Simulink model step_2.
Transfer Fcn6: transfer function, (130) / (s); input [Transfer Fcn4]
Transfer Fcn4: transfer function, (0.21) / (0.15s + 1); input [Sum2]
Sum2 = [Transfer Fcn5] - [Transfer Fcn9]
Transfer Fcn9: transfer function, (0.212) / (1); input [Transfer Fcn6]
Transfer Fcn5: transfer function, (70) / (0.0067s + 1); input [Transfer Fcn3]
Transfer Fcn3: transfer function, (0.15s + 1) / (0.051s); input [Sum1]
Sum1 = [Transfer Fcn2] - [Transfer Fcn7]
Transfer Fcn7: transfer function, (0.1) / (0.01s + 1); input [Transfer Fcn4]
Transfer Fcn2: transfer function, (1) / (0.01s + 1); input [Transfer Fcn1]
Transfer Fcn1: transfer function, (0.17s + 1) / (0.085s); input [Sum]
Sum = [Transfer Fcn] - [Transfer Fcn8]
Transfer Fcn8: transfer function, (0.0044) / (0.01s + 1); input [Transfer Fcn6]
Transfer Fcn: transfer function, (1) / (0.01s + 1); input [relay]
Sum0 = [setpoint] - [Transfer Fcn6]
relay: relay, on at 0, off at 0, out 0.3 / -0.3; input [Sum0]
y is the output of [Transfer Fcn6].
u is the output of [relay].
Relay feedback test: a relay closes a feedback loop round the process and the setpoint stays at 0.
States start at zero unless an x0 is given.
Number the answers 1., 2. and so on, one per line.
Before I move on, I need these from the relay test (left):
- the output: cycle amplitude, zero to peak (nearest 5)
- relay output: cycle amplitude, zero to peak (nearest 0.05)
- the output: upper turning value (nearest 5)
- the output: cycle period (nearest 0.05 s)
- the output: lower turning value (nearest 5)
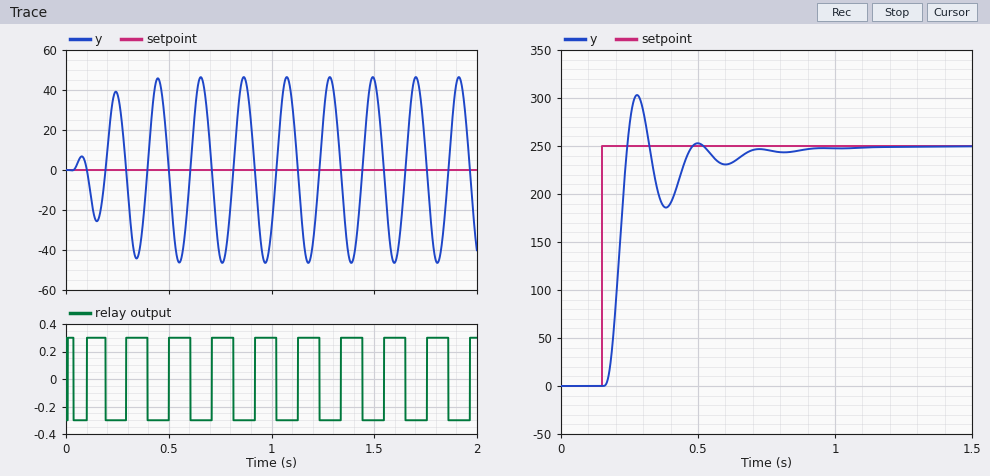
1. 45
2. 0.30
3. 45
4. 0.20 s
5. -45
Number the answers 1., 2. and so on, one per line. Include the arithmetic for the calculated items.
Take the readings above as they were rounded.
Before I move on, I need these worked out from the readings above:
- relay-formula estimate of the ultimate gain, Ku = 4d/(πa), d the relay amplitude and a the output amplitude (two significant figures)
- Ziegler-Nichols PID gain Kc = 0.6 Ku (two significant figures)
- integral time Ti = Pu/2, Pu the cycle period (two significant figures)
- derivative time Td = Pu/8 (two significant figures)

1. 4 × 0.3 / (π × 45) = 0.0085
2. 0.6 × 0.0085 = 0.0051
3. 0.2 / 2 = 0.10 s
4. 0.2 / 8 = 0.025 s
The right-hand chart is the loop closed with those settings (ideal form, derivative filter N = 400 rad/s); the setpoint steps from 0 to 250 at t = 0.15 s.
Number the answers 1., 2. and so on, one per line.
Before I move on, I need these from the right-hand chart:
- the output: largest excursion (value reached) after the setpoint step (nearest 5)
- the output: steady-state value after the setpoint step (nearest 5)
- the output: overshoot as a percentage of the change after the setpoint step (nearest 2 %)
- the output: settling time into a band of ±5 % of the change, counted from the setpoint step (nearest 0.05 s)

1. 305
2. 250
3. 22 %
4. 0.50 s
